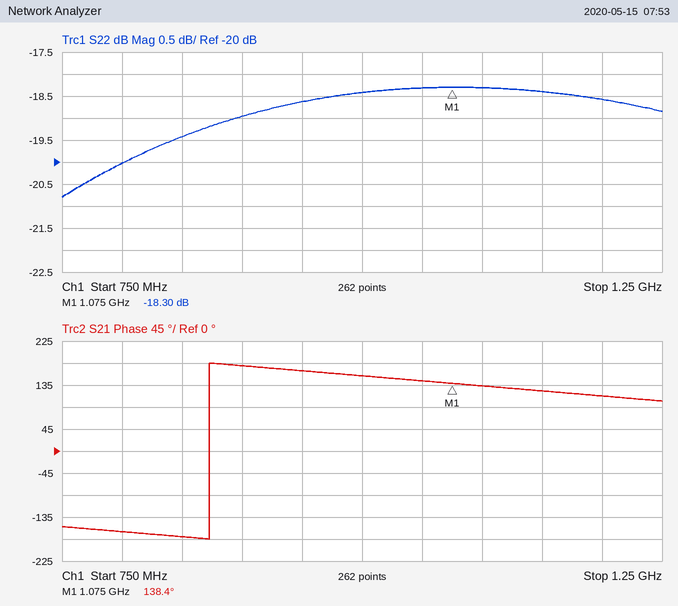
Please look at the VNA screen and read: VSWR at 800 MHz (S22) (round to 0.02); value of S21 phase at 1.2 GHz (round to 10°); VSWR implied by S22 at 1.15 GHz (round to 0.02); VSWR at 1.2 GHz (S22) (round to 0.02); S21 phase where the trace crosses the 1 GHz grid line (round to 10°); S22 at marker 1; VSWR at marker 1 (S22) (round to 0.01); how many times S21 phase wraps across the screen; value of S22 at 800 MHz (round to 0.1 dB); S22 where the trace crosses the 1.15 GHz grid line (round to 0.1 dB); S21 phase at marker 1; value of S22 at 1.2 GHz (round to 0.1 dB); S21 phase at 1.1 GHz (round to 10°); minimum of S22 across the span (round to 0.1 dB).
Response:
1.22
110°
1.28
1.26
150°
-18.30 dB
1.28
1
-20.0 dB
-18.4 dB
138.4°
-18.6 dB
130°
-20.8 dB
